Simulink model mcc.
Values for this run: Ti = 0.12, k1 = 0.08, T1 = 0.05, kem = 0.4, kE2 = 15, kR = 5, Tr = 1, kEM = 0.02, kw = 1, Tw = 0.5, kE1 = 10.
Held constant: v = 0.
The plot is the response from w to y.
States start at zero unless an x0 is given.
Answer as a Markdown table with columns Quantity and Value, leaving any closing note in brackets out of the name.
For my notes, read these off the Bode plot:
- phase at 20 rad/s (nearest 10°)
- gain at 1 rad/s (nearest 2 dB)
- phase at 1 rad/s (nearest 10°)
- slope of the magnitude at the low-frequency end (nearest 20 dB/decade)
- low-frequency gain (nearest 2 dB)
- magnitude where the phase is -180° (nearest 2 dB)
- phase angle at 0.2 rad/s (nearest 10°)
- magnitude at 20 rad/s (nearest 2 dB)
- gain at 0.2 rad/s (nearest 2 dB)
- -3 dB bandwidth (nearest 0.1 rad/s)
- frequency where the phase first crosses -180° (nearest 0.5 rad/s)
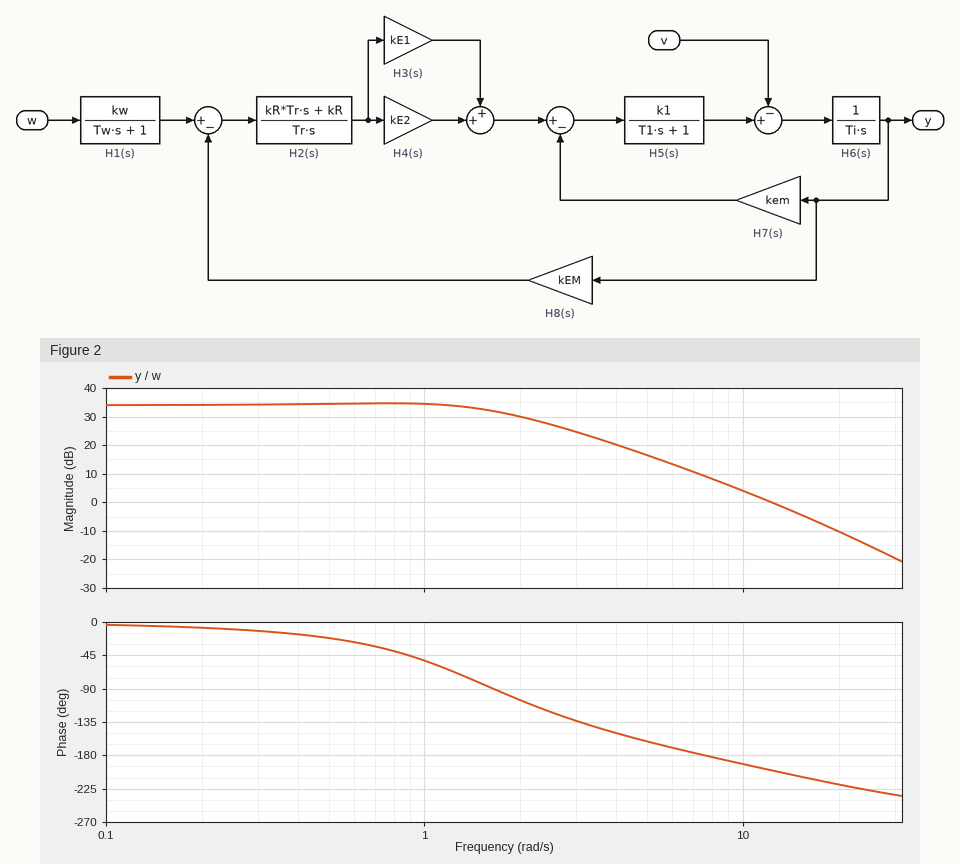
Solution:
| Quantity | Value |
|---|---|
| phase at 20 rad/s | -220° |
| gain at 1 rad/s | 34 dB |
| phase at 1 rad/s | -50° |
| slope of the magnitude at the low-frequency end | 0 dB/decade |
| low-frequency gain | 34 dB |
| magnitude where the phase is -180° | 10 dB |
| phase angle at 0.2 rad/s | -10° |
| magnitude at 20 rad/s | -10 dB |
| gain at 0.2 rad/s | 34 dB |
| -3 dB bandwidth | 1.8 rad/s |
| frequency where the phase first crosses -180° | 7.5 rad/s |
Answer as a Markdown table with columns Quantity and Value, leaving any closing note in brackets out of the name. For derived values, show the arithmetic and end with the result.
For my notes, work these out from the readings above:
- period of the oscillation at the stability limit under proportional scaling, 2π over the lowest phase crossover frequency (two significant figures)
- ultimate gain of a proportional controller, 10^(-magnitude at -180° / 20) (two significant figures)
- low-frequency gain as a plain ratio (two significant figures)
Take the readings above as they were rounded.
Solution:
| Quantity | Value |
|---|---|
| period of the oscillation at the stability limit under proportional scaling, 2π over the lowest phase crossover frequency | 2π / 7.5 = 0.84 s |
| ultimate gain of a proportional controller, 10^(-magnitude at -180° / 20) | 10^(-10 / 20) = 0.32 |
| low-frequency gain as a plain ratio | 10^(34 / 20) = 50 |
